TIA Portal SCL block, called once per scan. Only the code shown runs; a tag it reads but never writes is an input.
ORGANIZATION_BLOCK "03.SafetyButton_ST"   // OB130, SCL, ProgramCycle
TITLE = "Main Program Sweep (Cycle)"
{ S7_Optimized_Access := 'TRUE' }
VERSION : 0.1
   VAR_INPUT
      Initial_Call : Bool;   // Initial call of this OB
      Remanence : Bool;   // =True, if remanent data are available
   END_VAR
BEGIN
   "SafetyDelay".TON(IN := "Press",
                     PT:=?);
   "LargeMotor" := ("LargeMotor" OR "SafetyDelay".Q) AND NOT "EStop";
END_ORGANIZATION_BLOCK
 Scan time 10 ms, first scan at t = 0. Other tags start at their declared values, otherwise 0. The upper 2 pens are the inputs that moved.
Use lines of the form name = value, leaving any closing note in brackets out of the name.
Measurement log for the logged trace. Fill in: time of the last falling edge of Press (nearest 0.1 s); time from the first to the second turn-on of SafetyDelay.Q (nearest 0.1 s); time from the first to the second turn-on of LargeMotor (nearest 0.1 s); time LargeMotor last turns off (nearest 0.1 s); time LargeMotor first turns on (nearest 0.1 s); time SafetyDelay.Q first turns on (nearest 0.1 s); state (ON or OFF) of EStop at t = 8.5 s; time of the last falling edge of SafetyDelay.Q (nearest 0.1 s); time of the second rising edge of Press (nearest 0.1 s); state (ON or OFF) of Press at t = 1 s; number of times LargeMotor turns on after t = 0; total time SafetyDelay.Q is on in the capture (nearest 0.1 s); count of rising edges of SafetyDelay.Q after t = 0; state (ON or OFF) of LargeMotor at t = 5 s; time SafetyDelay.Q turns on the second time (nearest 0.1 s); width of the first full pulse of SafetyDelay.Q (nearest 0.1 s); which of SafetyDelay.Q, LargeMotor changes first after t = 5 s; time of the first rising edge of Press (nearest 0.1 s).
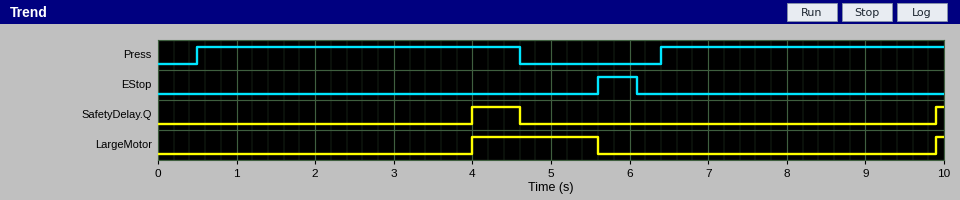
time of the last falling edge of Press = 4.6 s
time from the first to the second turn-on of SafetyDelay.Q = 5.9 s
time from the first to the second turn-on of LargeMotor = 5.9 s
time LargeMotor last turns off = 5.6 s
time LargeMotor first turns on = 4.0 s
time SafetyDelay.Q first turns on = 4.0 s
state (ON or OFF) of EStop at t = 8.5 s = OFF
time of the last falling edge of SafetyDelay.Q = 4.6 s
time of the second rising edge of Press = 6.4 s
state (ON or OFF) of Press at t = 1 s = ON
number of times LargeMotor turns on after t = 0 = 2
total time SafetyDelay.Q is on in the capture = 0.7 s
count of rising edges of SafetyDelay.Q after t = 0 = 2
state (ON or OFF) of LargeMotor at t = 5 s = ON
time SafetyDelay.Q turns on the second time = 9.9 s
width of the first full pulse of SafetyDelay.Q = 0.6 s
which of SafetyDelay.Q, LargeMotor changes first after t = 5 s = LargeMotor
time of the first rising edge of Press = 0.5 s
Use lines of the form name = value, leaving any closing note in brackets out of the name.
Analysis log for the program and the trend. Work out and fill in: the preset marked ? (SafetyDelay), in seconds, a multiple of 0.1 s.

the preset marked ? (SafetyDelay), in seconds, a multiple of 0.1 s = 3.5 s
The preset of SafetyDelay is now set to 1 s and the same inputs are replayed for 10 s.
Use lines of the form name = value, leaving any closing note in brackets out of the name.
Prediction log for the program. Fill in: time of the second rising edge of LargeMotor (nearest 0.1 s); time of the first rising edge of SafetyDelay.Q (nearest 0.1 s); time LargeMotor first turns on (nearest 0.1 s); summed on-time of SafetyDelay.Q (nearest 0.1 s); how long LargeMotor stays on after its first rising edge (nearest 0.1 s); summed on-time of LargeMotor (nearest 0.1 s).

time of the second rising edge of LargeMotor = 7.4 s
time of the first rising edge of SafetyDelay.Q = 1.5 s
time LargeMotor first turns on = 1.5 s
summed on-time of SafetyDelay.Q = 5.7 s
how long LargeMotor stays on after its first rising edge = 4.1 s
summed on-time of LargeMotor = 6.7 s
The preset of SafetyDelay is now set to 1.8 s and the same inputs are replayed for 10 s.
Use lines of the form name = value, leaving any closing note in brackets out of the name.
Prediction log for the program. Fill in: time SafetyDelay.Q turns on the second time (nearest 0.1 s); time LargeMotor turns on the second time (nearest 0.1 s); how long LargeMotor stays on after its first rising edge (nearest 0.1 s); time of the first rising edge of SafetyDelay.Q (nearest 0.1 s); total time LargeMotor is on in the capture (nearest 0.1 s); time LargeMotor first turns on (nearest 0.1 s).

time SafetyDelay.Q turns on the second time = 8.2 s
time LargeMotor turns on the second time = 8.2 s
how long LargeMotor stays on after its first rising edge = 3.3 s
time of the first rising edge of SafetyDelay.Q = 2.3 s
total time LargeMotor is on in the capture = 5.1 s
time LargeMotor first turns on = 2.3 s
